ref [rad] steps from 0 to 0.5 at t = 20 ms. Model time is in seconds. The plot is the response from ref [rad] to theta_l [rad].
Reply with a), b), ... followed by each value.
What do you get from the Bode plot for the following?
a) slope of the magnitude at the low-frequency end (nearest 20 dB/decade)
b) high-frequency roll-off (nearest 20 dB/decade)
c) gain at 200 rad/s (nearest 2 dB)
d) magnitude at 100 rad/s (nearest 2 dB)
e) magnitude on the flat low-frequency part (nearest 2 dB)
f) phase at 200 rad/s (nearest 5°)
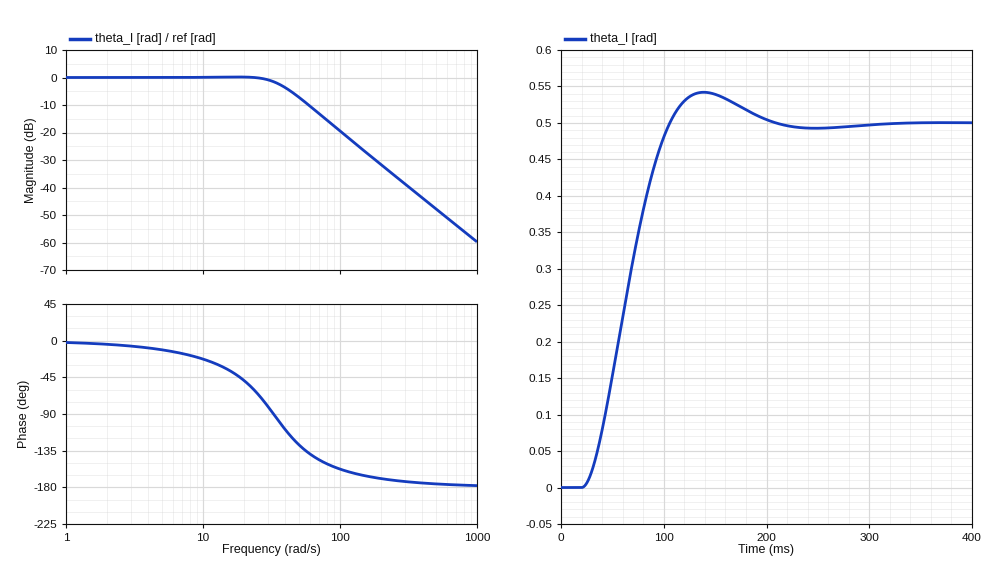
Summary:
a) 0 dB/decade
b) -40 dB/decade
c) -32 dB
d) -20 dB
e) 0 dB
f) -170°
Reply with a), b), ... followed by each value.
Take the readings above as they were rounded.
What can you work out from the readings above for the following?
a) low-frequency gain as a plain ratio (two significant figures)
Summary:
a) 1.0
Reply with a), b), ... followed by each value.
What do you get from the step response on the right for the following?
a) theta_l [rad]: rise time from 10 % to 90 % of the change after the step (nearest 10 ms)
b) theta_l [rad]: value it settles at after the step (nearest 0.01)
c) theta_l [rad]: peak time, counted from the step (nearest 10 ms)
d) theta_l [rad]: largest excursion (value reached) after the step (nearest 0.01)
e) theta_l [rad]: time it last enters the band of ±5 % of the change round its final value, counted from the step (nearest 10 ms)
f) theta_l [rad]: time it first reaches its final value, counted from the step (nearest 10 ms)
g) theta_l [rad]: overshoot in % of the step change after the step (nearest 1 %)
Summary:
a) 60 ms
b) 0.50
c) 120 ms
d) 0.54
e) 150 ms
f) 90 ms
g) 8 %
